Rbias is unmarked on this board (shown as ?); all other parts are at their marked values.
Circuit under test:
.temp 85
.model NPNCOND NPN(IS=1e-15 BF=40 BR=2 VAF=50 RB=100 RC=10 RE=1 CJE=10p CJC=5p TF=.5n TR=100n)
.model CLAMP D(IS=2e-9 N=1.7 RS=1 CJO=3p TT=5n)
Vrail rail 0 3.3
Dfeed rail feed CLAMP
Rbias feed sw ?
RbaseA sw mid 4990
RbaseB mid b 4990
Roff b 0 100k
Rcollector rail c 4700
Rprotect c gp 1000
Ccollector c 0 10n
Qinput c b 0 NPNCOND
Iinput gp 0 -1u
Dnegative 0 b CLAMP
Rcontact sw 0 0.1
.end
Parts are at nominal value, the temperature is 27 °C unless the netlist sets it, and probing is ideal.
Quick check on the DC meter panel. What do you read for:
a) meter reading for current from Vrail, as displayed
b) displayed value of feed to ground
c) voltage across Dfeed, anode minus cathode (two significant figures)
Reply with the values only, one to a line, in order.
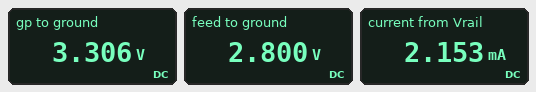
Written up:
2.153 mA
2.800 V
500 mV
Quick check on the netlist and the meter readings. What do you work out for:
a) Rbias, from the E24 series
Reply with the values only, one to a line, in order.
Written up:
1.3 kΩ
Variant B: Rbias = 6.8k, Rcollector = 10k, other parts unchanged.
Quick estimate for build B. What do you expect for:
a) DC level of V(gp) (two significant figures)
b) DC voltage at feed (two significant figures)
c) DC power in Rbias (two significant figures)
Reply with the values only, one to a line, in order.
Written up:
3.3 V
2.9 V
1.2 mW
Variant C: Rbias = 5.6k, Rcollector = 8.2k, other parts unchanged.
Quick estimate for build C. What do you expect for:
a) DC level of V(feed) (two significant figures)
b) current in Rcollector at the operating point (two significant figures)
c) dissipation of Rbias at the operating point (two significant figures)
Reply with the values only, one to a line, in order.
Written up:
2.9 V
1.0 µA
1.5 mW
